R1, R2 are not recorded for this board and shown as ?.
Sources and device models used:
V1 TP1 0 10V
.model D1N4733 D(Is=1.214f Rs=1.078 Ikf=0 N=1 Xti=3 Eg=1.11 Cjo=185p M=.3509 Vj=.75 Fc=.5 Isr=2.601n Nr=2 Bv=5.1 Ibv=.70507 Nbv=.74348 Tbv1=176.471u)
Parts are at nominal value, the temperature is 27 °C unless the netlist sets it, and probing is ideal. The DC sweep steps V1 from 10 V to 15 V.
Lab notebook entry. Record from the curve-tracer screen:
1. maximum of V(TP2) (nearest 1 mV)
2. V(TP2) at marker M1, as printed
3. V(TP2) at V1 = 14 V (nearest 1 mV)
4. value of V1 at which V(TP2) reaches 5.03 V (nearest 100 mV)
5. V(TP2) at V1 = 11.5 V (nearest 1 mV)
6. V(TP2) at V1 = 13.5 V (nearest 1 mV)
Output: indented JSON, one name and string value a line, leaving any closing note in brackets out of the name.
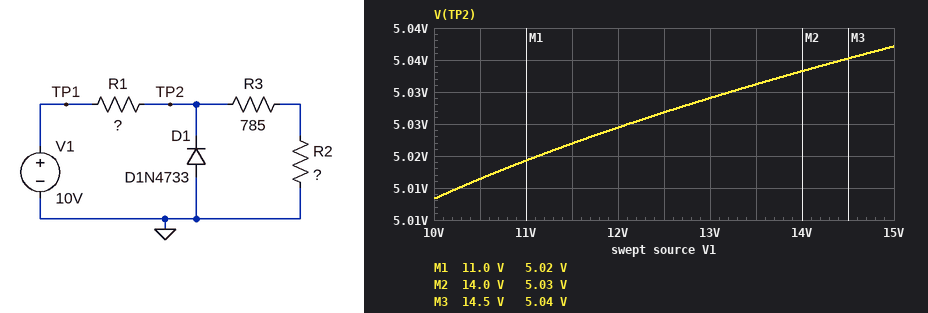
{
  "maximum of V(TP2)": "5.037 V",
  "V(TP2) at marker M1, as printed": "5.02 V",
  "V(TP2) at V1 = 14 V": "5.033 V",
  "value of V1 at which V(TP2) reaches 5.03 V": "12.1 V",
  "V(TP2) at V1 = 11.5 V": "5.022 V",
  "V(TP2) at V1 = 13.5 V": "5.031 V"
}
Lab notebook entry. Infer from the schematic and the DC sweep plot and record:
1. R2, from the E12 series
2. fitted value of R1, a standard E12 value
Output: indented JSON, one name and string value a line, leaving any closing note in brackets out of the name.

{
  "R2, from the E12 series": "2.2 kΩ",
  "fitted value of R1, a standard E12 value": "680 Ω"
}
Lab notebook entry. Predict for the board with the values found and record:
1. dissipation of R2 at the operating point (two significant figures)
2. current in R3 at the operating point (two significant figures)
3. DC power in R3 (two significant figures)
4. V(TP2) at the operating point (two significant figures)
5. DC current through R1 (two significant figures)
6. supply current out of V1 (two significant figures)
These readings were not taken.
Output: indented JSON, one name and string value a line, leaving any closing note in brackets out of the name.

{
  "dissipation of R2 at the operating point": "6.2 mW",
  "current in R3 at the operating point": "1.7 mA",
  "DC power in R3": "2.2 mW",
  "V(TP2) at the operating point": "5.0 V",
  "DC current through R1": "7.3 mA",
  "supply current out of V1": "7.3 mA"
}
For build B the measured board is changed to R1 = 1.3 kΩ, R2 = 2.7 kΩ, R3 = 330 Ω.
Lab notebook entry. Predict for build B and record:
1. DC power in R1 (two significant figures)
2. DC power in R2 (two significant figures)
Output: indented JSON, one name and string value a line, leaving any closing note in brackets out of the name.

{
  "DC power in R1": "19 mW",
  "DC power in R2": "7.3 mW"
}
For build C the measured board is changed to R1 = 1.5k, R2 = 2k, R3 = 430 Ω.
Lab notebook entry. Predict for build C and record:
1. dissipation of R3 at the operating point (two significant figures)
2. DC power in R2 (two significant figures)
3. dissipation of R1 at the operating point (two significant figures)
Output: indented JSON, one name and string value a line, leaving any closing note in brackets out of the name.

{
  "dissipation of R3 at the operating point": "1.8 mW",
  "DC power in R2": "8.4 mW",
  "dissipation of R1 at the operating point": "17 mW"
}
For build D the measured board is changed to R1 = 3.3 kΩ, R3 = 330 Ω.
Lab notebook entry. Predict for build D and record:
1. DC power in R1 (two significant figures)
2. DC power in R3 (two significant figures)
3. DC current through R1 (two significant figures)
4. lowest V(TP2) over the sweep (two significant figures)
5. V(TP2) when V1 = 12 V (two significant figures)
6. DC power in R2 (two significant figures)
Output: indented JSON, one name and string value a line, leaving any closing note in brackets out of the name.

{
  "DC power in R1": "9.7 mW",
  "DC power in R3": "970 µW",
  "DC current through R1": "1.7 mA",
  "lowest V(TP2) over the sweep": "4.3 V",
  "V(TP2) when V1 = 12 V": "4.9 V",
  "DC power in R2": "6.5 mW"
}
